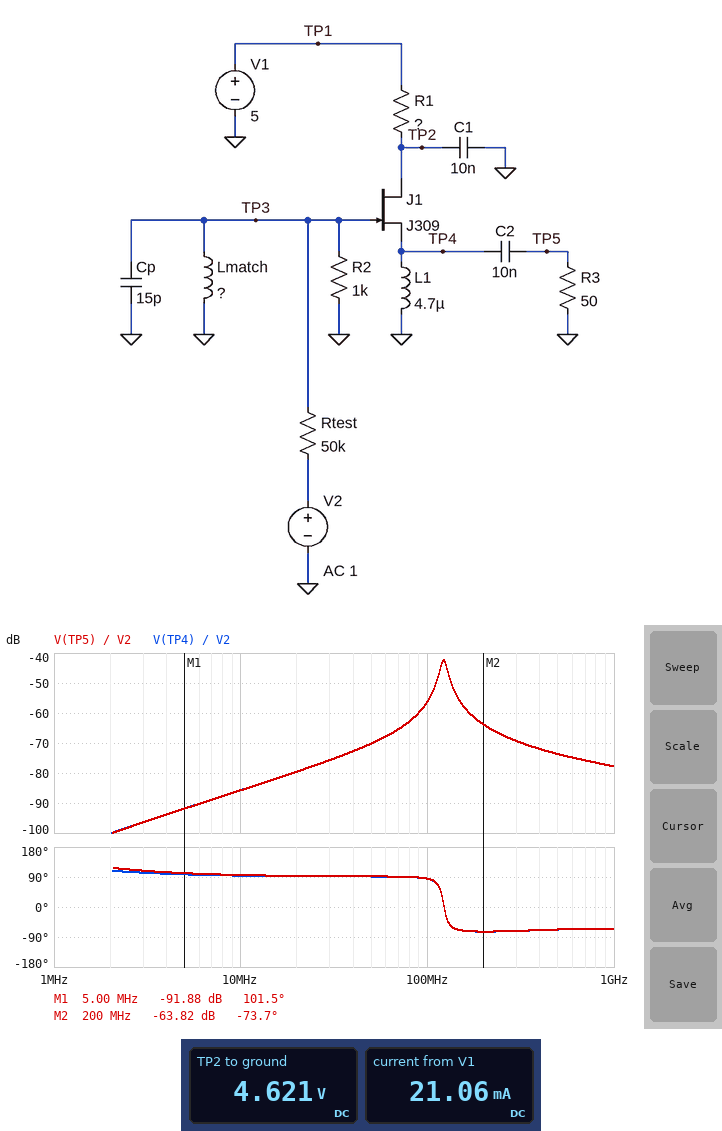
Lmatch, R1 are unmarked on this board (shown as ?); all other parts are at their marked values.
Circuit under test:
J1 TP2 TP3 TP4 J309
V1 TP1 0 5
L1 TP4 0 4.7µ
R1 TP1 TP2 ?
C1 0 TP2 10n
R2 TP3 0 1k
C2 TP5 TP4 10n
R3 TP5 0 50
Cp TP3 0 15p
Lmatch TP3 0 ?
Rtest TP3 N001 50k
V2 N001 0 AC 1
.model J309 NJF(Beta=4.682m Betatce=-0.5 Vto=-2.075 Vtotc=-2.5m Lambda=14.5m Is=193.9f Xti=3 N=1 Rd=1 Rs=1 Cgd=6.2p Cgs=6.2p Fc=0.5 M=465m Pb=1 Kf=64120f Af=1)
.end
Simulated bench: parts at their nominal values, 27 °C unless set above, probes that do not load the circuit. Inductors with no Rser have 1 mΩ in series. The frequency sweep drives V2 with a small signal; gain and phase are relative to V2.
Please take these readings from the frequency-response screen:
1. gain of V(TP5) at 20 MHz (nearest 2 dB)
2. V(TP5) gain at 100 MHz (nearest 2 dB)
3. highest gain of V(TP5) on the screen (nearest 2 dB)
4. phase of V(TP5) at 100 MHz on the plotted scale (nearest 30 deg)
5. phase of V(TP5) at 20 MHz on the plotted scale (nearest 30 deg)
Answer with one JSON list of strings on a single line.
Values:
["-80 dB", "-56 dB", "-42 dB", "90 deg", "90 deg"]
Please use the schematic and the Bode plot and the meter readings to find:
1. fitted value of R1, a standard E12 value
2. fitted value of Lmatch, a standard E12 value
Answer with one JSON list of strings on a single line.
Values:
["18 Ω", "82 nH"]
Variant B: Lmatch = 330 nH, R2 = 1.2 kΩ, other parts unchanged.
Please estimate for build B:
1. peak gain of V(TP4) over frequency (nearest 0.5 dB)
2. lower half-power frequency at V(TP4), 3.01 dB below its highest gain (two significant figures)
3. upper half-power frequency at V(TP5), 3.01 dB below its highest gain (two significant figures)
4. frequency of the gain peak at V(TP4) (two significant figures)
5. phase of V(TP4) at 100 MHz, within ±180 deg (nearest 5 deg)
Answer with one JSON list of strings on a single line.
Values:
["-39.5 dB", "57 MHz", "65 MHz", "61 MHz", "-75 deg"]
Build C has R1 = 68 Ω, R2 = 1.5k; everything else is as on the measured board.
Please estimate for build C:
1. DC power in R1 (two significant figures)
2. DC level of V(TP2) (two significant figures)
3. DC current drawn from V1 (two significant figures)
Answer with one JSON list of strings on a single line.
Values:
["29 mW", "3.6 V", "21 mA"]
